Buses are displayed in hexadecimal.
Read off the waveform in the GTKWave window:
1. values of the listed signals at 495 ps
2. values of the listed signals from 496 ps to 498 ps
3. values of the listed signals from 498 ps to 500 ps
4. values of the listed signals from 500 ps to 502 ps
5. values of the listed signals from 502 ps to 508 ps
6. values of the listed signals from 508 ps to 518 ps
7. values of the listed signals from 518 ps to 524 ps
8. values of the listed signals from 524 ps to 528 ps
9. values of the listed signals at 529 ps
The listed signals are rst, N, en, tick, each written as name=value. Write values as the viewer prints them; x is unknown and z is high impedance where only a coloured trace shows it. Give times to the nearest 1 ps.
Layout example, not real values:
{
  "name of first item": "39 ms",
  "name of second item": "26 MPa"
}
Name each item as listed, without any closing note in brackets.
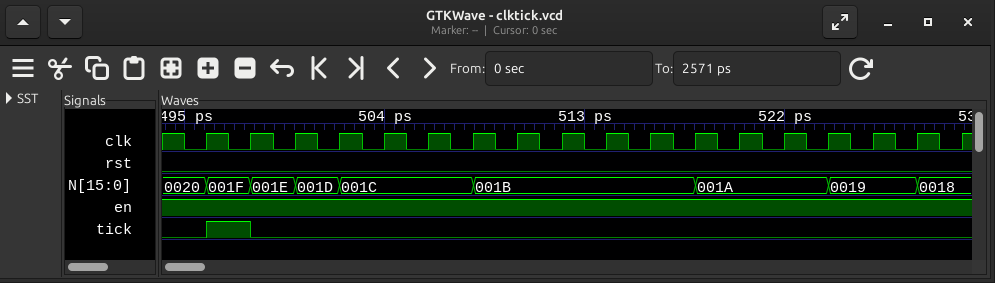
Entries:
{
  "values of the listed signals at 495 ps": "rst=0, N=0020, en=1, tick=0",
  "values of the listed signals from 496 ps to 498 ps": "rst=0, N=001F, en=1, tick=1",
  "values of the listed signals from 498 ps to 500 ps": "rst=0, N=001E, en=1, tick=0",
  "values of the listed signals from 500 ps to 502 ps": "rst=0, N=001D, en=1, tick=0",
  "values of the listed signals from 502 ps to 508 ps": "rst=0, N=001C, en=1, tick=0",
  "values of the listed signals from 508 ps to 518 ps": "rst=0, N=001B, en=1, tick=0",
  "values of the listed signals from 518 ps to 524 ps": "rst=0, N=001A, en=1, tick=0",
  "values of the listed signals from 524 ps to 528 ps": "rst=0, N=0019, en=1, tick=0",
  "values of the listed signals at 529 ps": "rst=0, N=0018, en=1, tick=0"
}
